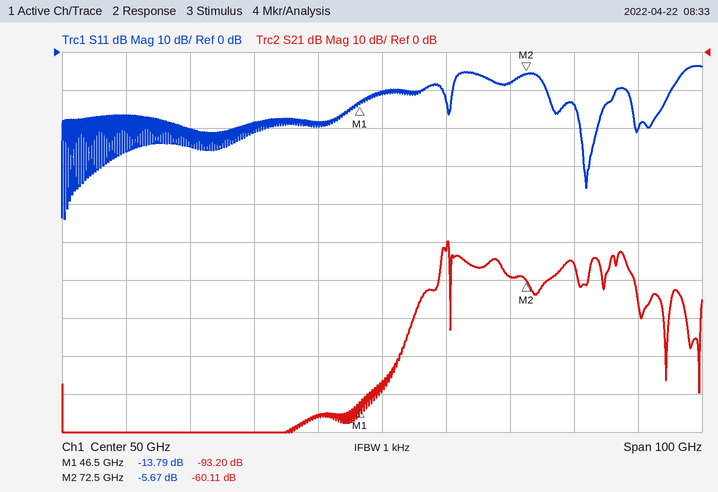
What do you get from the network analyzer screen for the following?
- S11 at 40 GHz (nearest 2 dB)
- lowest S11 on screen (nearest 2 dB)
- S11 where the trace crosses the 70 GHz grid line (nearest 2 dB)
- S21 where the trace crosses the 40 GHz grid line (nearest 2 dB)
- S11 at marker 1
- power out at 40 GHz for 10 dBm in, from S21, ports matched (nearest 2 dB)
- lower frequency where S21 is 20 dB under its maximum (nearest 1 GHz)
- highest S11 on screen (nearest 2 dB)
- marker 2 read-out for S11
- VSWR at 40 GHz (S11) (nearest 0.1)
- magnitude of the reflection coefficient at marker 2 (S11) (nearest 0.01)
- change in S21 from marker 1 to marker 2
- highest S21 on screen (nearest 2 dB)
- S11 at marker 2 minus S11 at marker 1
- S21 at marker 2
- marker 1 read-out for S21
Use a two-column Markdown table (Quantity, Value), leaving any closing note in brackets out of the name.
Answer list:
| Quantity | Value |
|---|---|
| S11 at 40 GHz | -18 dB |
| lowest S11 on screen | -44 dB |
| S11 where the trace crosses the 70 GHz grid line | -8 dB |
| S21 where the trace crosses the 40 GHz grid line | -96 dB |
| S11 at marker 1 | -13.79 dB |
| power out at 40 GHz for 10 dBm in, from S21, ports matched | -86 dBm |
| lower frequency where S21 is 20 dB under its maximum | 55 GHz |
| highest S11 on screen | -4 dB |
| marker 2 read-out for S11 | -5.67 dB |
| VSWR at 40 GHz (S11) | 1.3 |
| magnitude of the reflection coefficient at marker 2 (S11) | 0.52 |
| change in S21 from marker 1 to marker 2 | 33.09 dB |
| highest S21 on screen | -50 dB |
| S11 at marker 2 minus S11 at marker 1 | 8.12 dB |
| S21 at marker 2 | -60.11 dB |
| marker 1 read-out for S21 | -93.20 dB |
